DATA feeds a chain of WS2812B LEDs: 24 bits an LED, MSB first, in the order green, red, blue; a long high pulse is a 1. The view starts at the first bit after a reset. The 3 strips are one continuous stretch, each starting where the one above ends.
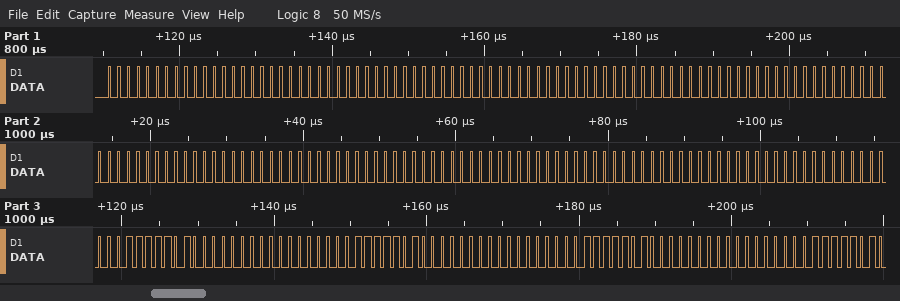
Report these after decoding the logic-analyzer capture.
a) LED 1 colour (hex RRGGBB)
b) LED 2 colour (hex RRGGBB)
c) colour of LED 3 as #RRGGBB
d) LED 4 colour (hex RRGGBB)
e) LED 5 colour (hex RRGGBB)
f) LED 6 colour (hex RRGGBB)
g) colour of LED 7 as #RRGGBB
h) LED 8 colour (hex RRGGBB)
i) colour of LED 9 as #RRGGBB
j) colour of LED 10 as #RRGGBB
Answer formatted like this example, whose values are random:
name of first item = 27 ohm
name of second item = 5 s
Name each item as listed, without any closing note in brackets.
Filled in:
LED 1 colour = #000000
LED 2 colour = #000000
colour of LED 3 as #RRGGBB = #000000
LED 4 colour = #000000
LED 5 colour = #000000
LED 6 colour = #000000
colour of LED 7 as #RRGGBB = #000000
LED 8 colour = #00FA00
colour of LED 9 as #RRGGBB = #00FA00
colour of LED 10 as #RRGGBB = #00FA00
